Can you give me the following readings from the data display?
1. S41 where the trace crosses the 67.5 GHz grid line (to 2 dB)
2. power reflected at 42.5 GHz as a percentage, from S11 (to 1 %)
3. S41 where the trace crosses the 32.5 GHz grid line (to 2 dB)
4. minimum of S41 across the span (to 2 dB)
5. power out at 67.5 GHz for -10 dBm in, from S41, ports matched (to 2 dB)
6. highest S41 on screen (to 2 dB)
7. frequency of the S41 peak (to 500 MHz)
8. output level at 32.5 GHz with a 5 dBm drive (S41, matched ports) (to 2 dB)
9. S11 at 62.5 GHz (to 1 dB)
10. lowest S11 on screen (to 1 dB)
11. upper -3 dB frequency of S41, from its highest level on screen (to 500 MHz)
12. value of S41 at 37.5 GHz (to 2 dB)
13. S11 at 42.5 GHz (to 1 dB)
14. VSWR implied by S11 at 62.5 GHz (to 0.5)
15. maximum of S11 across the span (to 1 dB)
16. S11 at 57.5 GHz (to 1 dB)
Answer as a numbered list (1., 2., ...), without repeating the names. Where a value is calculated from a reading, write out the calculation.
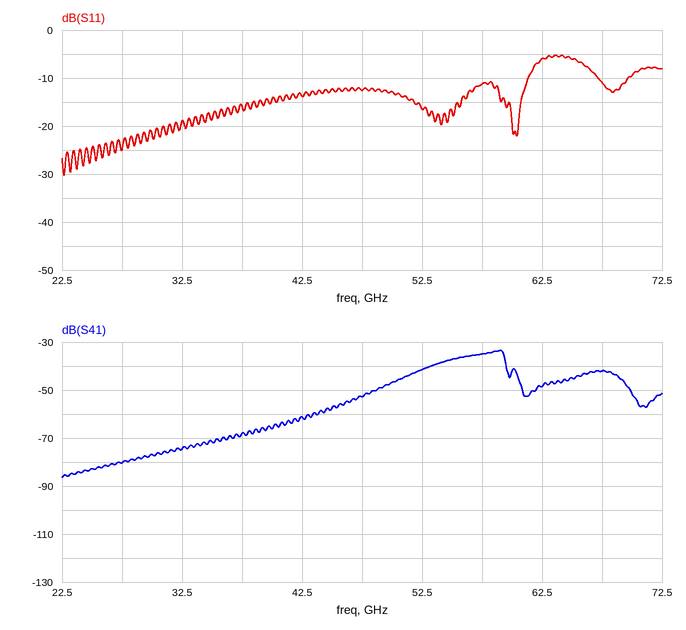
1. -42 dB
2. 10^(-14/10) ≈ 4 %
3. -74 dB
4. -86 dB
5. -10 dBm + (-42 dB) = -52 dBm
6. -34 dB
7. 59.0 GHz
8. 5 dBm + (-74 dB) = -70 dBm
9. -6 dB
10. -30 dB
11. 59.5 GHz
12. -68 dB
13. -14 dB
14. |Γ| = 10^(-6/20) = 0.5012; VSWR = (1 + 0.5012)/(1 − 0.5012) ≈ 3.0
15. -5 dB
16. -11 dB
